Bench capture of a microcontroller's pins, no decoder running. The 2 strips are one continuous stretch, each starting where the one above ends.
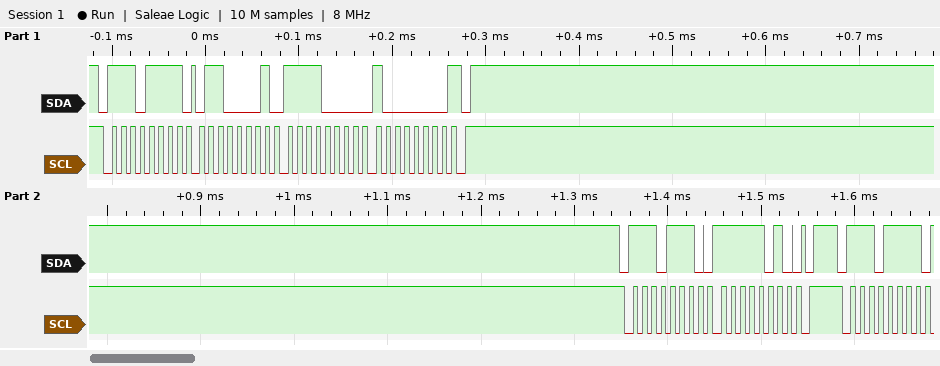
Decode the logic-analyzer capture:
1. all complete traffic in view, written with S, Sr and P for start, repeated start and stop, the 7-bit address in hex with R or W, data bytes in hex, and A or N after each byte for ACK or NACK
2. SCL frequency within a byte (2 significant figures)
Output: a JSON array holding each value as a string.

["S 77R A 61 A F0 A 80 N P S 77W A FA A P S 77R A", "100 kHz"]
